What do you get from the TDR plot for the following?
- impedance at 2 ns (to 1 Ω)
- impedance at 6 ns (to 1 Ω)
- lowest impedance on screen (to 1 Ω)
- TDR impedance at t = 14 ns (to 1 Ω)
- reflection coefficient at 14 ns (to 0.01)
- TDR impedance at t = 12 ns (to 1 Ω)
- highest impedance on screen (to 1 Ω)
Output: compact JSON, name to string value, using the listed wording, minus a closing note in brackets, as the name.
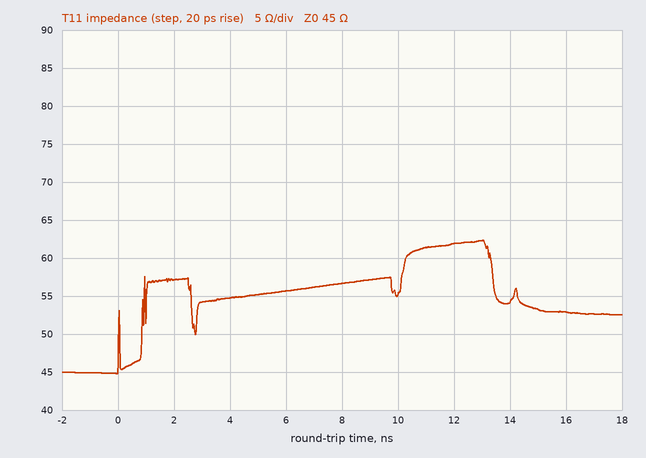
{"impedance at 2 ns": "57 Ω", "impedance at 6 ns": "56 Ω", "lowest impedance on screen": "45 Ω", "TDR impedance at t = 14 ns": "54 Ω", "reflection coefficient at 14 ns": "+0.09", "TDR impedance at t = 12 ns": "62 Ω", "highest impedance on screen": "62 Ω"}
